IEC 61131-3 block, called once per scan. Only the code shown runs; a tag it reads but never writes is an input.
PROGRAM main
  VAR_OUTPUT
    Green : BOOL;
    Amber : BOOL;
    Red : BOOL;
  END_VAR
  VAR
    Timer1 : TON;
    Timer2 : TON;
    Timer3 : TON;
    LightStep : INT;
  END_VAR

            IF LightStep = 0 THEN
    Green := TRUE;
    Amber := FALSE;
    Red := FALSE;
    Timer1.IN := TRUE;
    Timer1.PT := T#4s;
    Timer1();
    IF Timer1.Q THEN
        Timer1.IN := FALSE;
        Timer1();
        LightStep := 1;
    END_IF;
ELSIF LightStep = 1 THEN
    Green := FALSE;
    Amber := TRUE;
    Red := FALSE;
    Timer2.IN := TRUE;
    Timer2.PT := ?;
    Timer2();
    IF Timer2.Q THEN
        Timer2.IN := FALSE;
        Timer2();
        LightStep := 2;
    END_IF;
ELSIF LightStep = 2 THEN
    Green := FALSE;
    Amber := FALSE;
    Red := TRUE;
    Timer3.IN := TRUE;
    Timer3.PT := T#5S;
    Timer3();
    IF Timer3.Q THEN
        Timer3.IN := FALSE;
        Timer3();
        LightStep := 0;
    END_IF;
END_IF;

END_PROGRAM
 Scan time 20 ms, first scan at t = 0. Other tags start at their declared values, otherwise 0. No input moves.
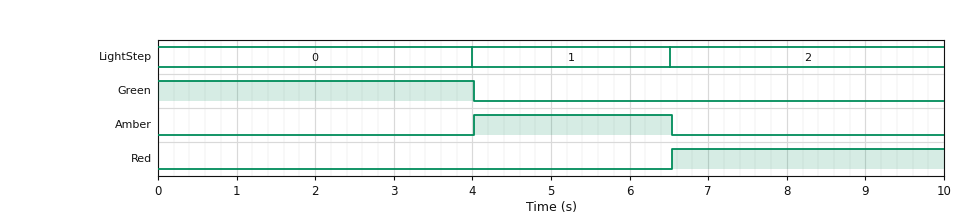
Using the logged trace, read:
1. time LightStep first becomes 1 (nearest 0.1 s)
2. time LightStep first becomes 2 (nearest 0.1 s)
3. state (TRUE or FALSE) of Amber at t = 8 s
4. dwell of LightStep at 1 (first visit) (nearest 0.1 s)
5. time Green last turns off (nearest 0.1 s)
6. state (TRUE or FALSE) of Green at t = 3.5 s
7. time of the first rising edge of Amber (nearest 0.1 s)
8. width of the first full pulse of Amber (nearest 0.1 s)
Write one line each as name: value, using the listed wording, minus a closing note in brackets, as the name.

time LightStep first becomes 1: 4.0 s
time LightStep first becomes 2: 6.5 s
state (TRUE or FALSE) of Amber at t = 8 s: FALSE
dwell of LightStep at 1 (first visit): 2.5 s
time Green last turns off: 4.0 s
state (TRUE or FALSE) of Green at t = 3.5 s: TRUE
time of the first rising edge of Amber: 4.0 s
width of the first full pulse of Amber: 2.5 s
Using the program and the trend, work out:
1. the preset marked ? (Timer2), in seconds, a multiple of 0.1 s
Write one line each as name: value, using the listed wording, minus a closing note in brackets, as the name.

the preset marked ? (Timer2), in seconds, a multiple of 0.1 s: 2.5 s
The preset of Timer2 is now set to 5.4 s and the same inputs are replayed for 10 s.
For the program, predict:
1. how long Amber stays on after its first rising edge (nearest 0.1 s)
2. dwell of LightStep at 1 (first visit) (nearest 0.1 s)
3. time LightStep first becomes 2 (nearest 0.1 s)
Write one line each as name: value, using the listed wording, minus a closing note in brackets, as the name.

how long Amber stays on after its first rising edge: 5.4 s
dwell of LightStep at 1 (first visit): 5.4 s
time LightStep first becomes 2: 9.4 s
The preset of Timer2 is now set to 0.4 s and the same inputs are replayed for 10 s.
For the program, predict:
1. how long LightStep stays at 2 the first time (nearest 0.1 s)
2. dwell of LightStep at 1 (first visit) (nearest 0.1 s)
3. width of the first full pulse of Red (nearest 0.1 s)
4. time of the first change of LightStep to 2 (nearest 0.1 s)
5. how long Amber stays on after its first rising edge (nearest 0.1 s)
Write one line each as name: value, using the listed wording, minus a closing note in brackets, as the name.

how long LightStep stays at 2 the first time: 5.0 s
dwell of LightStep at 1 (first visit): 0.4 s
width of the first full pulse of Red: 5.0 s
time of the first change of LightStep to 2: 4.4 s
how long Amber stays on after its first rising edge: 0.4 s
